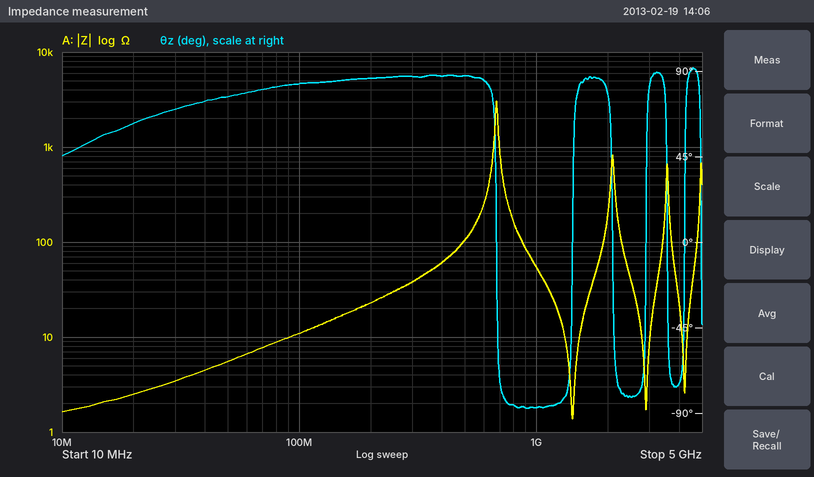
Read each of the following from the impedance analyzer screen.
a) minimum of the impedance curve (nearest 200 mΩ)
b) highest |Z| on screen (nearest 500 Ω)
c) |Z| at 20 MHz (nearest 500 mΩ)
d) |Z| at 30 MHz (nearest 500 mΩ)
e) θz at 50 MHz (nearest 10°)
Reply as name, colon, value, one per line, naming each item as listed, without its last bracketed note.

minimum of the impedance curve: 1.4 Ω
highest |Z| on screen: 3.0 kΩ
|Z| at 20 MHz: 2.5 Ω
|Z| at 30 MHz: 3.5 Ω
θz at 50 MHz: 80°
